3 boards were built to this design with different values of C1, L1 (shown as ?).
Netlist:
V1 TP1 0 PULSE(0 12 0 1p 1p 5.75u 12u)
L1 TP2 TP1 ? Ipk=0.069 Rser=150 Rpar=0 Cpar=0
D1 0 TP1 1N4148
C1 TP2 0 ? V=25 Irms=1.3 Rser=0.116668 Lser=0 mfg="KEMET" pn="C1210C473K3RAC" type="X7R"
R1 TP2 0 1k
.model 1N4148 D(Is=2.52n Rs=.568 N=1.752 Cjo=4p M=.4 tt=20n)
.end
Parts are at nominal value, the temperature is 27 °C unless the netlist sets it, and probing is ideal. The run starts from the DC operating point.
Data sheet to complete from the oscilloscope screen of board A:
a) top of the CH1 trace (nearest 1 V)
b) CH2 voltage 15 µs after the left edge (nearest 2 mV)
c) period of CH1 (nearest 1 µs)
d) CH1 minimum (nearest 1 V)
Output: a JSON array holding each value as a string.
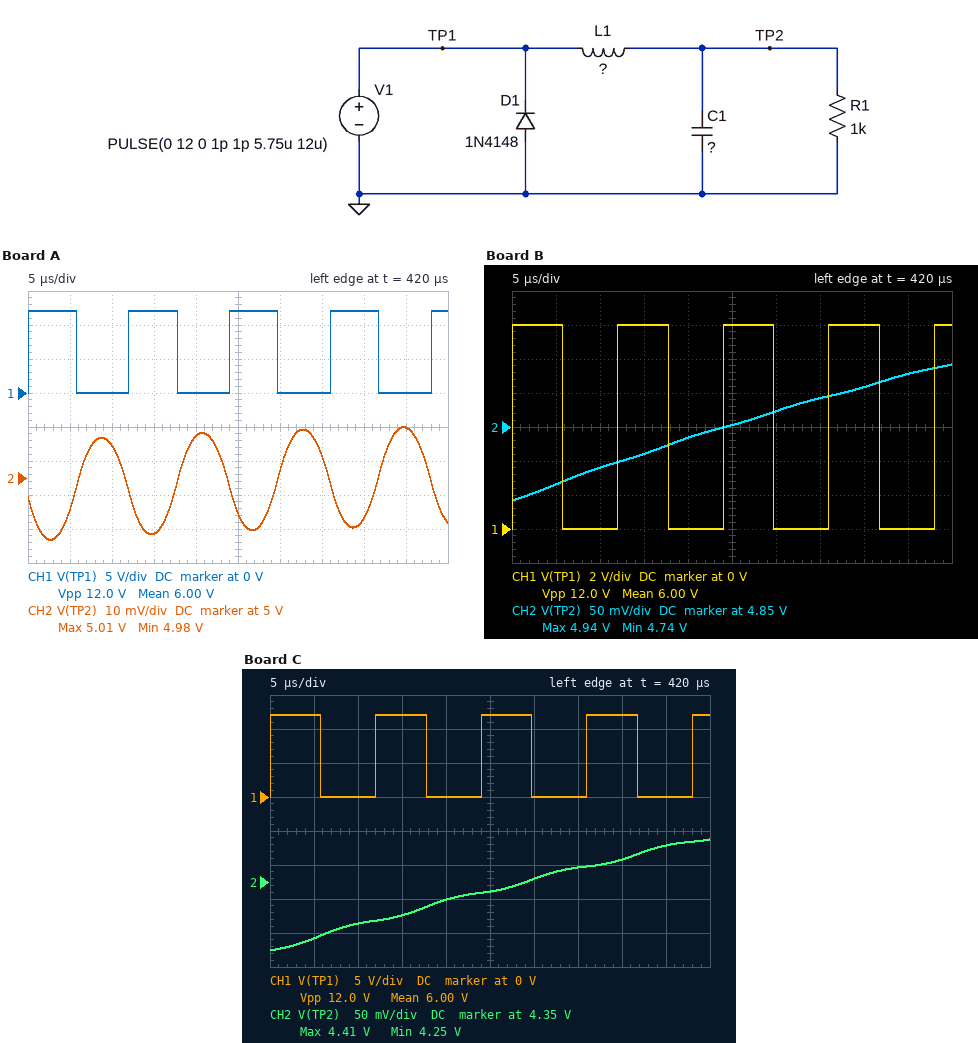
["12 V", "4.984 V", "12 µs", "0 V"]
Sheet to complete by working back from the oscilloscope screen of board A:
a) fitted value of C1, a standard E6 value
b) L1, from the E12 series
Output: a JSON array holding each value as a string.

["33 nF", "56 mH"]
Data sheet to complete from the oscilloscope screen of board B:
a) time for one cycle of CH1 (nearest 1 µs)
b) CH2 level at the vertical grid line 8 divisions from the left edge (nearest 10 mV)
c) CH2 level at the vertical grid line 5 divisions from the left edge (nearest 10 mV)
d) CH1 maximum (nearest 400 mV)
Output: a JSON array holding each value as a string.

["12 µs", "4.91 V", "4.85 V", "12.0 V"]
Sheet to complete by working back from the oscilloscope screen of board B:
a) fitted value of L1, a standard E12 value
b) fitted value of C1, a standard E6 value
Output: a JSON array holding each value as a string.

["220 mH", "100 nF"]
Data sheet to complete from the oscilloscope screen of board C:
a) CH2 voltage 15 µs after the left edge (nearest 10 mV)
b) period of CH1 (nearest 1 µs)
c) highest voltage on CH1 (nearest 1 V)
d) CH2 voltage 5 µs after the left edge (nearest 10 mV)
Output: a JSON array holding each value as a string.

["4.30 V", "12 µs", "12 V", "4.27 V"]
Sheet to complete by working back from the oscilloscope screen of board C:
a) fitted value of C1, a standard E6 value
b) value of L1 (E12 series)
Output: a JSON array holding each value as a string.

["33 nF", "270 mH"]
